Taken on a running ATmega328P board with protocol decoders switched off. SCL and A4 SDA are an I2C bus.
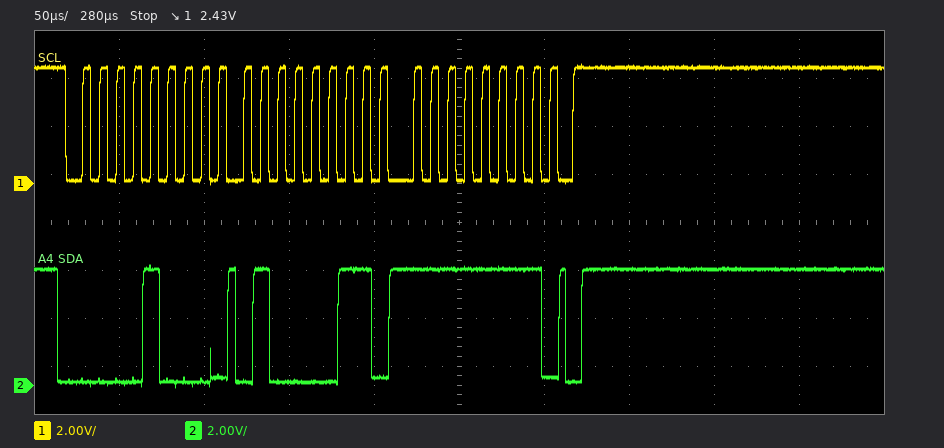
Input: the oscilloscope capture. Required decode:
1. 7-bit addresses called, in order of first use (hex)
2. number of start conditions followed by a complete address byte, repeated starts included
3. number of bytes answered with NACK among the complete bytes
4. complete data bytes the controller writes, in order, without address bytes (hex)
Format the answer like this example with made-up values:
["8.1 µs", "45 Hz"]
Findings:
["0x04", "1", "0", "43 FF"]
